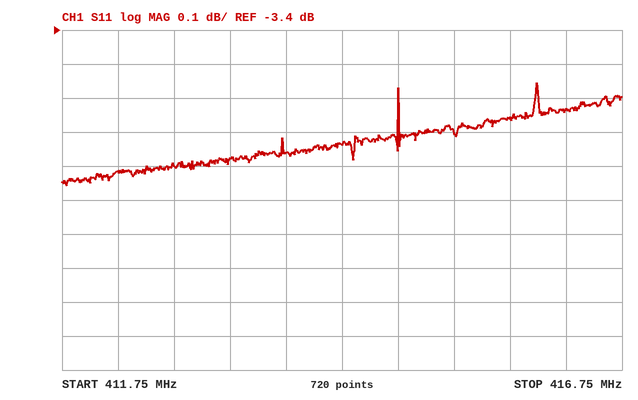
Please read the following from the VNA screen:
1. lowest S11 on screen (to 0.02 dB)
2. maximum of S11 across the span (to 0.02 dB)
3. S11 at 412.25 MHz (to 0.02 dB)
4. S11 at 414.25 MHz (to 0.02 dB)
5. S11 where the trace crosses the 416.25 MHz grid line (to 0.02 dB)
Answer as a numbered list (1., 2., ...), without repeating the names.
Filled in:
1. -3.86 dB
2. -3.56 dB
3. -3.82 dB
4. -3.74 dB
5. -3.64 dB
